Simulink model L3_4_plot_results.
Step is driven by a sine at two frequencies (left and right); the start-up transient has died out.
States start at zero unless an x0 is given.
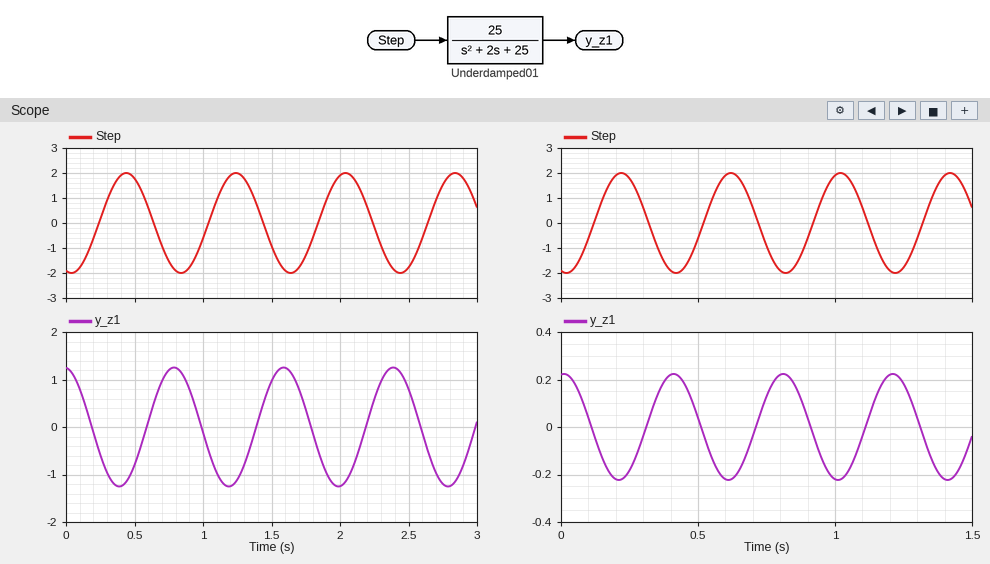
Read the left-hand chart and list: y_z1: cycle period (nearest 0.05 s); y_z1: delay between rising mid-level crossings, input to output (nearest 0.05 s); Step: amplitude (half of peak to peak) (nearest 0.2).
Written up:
0.80 s
0.35 s
2.0
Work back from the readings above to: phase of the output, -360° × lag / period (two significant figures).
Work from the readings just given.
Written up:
-160°
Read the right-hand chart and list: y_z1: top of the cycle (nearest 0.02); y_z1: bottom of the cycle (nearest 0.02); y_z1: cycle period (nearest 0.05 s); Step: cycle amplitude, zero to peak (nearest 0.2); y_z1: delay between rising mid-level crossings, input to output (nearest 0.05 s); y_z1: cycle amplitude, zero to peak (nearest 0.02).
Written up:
0.22
-0.22
0.40 s
2.0
0.20 s
0.22
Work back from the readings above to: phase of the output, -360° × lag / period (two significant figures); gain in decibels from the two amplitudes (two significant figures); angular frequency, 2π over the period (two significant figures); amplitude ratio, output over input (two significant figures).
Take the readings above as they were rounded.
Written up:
-180°
-19 dB
16 rad/s
0.11
